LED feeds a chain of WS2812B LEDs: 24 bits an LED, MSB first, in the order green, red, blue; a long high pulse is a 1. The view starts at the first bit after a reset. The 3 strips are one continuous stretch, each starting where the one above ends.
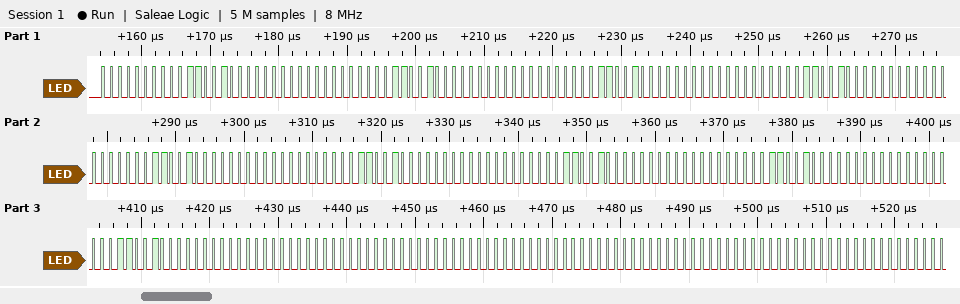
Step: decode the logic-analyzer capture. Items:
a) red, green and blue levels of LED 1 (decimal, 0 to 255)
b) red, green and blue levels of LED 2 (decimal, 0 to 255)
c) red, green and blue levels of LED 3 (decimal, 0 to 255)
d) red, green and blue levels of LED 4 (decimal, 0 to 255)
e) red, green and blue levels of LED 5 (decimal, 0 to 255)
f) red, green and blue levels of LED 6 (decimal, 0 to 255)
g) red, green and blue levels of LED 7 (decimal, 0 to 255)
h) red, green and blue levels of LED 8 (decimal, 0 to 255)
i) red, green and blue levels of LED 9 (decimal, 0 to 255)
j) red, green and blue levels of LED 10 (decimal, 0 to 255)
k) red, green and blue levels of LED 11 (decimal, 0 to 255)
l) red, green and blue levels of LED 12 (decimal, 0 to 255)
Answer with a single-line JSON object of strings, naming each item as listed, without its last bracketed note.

{"red, green and blue levels of LED 1": "50, 0, 0", "red, green and blue levels of LED 2": "50, 0, 0", "red, green and blue levels of LED 3": "50, 0, 0", "red, green and blue levels of LED 4": "50, 0, 0", "red, green and blue levels of LED 5": "50, 0, 0", "red, green and blue levels of LED 6": "50, 0, 0", "red, green and blue levels of LED 7": "50, 0, 0", "red, green and blue levels of LED 8": "50, 0, 0", "red, green and blue levels of LED 9": "50, 0, 0", "red, green and blue levels of LED 10": "0, 0, 0", "red, green and blue levels of LED 11": "0, 0, 0", "red, green and blue levels of LED 12": "0, 0, 0"}
